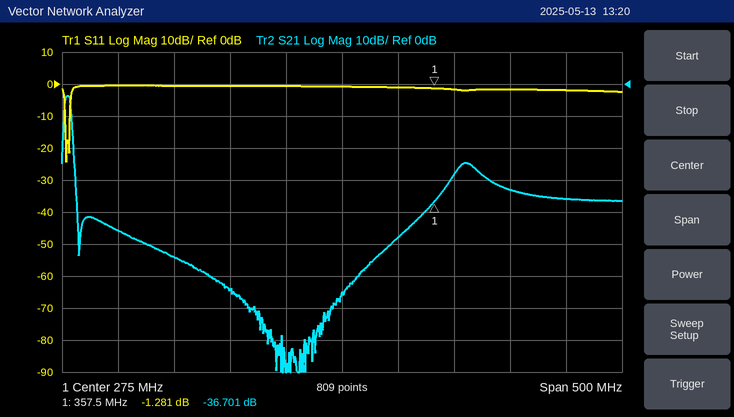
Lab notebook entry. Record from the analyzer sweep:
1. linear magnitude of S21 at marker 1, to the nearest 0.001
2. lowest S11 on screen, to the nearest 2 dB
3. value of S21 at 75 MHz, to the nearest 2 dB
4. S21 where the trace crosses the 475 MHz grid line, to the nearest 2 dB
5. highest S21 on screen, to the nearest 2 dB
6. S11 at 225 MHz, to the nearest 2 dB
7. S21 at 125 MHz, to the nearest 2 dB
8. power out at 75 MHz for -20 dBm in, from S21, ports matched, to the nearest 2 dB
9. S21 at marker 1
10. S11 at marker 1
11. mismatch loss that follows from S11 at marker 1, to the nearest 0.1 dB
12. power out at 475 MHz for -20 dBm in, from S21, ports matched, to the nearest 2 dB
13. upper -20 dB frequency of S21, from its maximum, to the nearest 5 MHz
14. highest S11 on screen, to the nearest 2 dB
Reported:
0.015
-24 dB
-46 dB
-36 dB
-4 dB
0 dB
-54 dB
-66 dBm
-36.701 dB
-1.281 dB
5.9 dB
-56 dBm
35 MHz
0 dB
